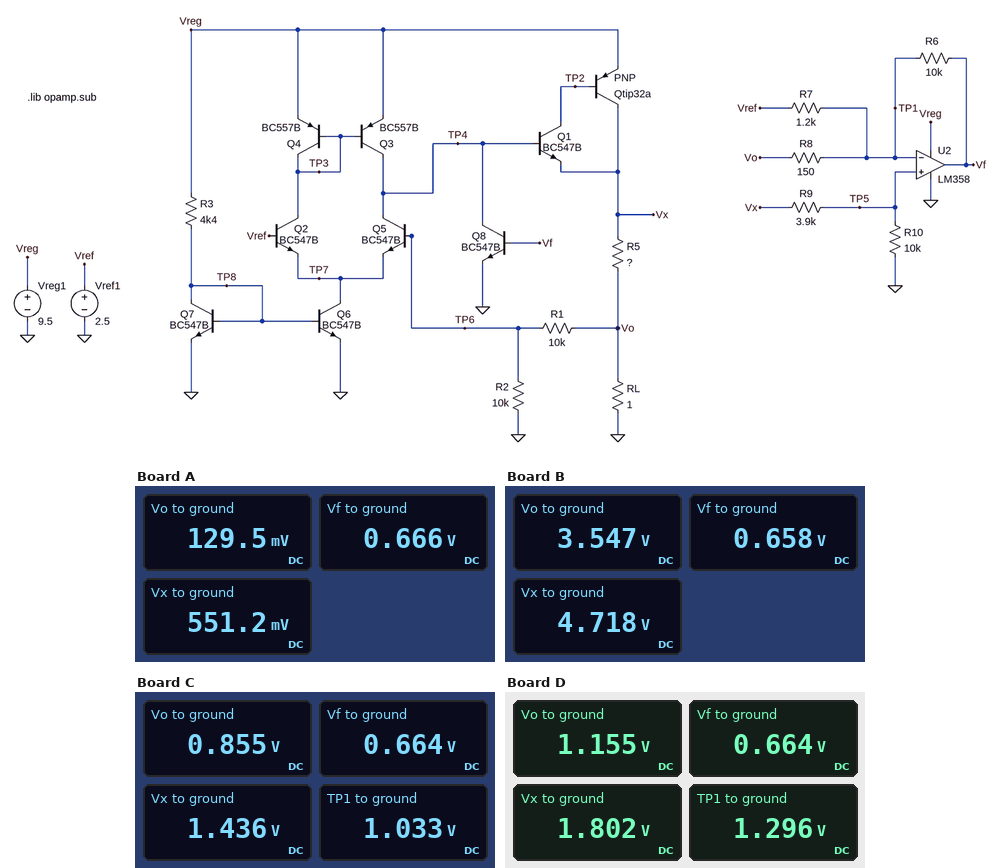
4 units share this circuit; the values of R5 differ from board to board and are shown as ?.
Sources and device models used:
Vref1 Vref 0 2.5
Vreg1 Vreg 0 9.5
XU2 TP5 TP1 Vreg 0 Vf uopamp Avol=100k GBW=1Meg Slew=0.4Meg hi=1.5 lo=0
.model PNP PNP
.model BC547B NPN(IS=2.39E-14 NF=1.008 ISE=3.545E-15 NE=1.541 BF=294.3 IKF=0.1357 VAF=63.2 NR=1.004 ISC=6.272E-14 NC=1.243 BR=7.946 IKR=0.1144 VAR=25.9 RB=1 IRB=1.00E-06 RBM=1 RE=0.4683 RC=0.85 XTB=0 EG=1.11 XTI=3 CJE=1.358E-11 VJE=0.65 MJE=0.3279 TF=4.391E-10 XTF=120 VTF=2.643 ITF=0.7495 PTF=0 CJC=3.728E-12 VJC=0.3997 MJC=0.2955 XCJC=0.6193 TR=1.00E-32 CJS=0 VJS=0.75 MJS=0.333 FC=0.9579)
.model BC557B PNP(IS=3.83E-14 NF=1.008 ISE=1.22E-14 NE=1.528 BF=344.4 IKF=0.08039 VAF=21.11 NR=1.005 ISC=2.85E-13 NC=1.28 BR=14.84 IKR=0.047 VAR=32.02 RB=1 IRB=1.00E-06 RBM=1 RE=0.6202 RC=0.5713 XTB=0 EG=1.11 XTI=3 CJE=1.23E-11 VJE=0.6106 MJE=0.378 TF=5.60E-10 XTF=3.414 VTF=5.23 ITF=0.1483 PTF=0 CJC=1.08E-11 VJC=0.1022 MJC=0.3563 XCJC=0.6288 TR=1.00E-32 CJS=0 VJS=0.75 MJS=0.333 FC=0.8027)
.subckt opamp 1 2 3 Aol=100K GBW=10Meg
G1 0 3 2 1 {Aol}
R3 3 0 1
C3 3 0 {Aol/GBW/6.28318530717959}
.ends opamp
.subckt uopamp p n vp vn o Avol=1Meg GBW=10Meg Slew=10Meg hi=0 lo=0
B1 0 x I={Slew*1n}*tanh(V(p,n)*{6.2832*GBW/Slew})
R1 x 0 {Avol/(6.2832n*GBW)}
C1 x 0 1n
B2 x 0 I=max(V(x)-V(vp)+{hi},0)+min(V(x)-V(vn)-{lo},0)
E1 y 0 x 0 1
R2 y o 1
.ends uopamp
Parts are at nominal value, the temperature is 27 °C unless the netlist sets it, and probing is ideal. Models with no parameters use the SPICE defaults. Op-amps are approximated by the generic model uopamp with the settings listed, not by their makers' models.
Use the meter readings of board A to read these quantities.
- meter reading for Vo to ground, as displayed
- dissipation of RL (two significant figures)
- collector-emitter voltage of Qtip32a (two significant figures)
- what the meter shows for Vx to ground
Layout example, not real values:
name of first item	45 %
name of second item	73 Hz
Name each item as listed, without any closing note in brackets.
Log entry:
meter reading for Vo to ground, as displayed	129.5 mV
dissipation of RL	17 mW
collector-emitter voltage of Qtip32a	-8.9 V
what the meter shows for Vx to ground	551.2 mV
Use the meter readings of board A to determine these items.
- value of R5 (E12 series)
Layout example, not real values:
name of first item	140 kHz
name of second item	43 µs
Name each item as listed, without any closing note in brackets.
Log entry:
value of R5	3.3 Ω
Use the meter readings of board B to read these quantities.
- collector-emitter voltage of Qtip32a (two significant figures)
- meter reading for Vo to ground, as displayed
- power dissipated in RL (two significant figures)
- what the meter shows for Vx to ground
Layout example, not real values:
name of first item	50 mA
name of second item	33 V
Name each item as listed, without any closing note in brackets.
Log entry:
collector-emitter voltage of Qtip32a	-4.8 V
meter reading for Vo to ground, as displayed	3.547 V
power dissipated in RL	13 W
what the meter shows for Vx to ground	4.718 V
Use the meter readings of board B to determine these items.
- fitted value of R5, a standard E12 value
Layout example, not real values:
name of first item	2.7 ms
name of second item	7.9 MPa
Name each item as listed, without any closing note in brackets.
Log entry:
fitted value of R5, a standard E12 value	0.33 Ω
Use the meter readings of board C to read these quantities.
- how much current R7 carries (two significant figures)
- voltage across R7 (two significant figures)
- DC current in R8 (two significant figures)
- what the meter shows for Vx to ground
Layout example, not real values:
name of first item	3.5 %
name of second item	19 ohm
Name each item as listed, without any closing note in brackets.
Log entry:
how much current R7 carries	1.2 mA
voltage across R7	1.5 V
DC current in R8	1.2 mA
what the meter shows for Vx to ground	1.436 V
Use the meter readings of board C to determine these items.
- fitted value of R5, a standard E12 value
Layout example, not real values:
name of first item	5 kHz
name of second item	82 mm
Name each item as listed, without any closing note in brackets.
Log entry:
fitted value of R5, a standard E12 value	0.68 Ω
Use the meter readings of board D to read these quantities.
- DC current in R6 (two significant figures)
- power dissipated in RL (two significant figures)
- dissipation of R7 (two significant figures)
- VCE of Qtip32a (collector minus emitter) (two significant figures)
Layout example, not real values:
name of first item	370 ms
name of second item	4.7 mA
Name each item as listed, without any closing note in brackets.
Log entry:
DC current in R6	63 µA
power dissipated in RL	1.3 W
dissipation of R7	1.2 mW
VCE of Qtip32a (collector minus emitter)	-7.7 V
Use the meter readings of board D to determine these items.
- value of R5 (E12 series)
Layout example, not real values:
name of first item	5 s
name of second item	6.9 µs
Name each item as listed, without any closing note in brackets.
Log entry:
value of R5	0.56 Ω
